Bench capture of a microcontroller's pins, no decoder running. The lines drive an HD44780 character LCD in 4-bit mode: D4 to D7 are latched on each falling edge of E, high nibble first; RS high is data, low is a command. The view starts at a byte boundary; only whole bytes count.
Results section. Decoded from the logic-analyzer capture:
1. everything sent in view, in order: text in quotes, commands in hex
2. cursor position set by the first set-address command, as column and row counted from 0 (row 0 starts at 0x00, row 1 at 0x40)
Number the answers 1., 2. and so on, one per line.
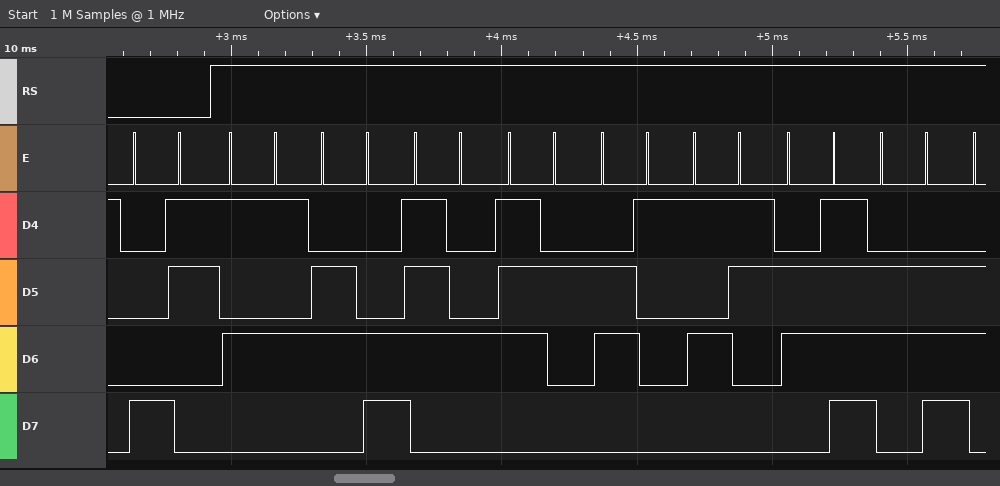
1. 0x83 "UltraSon"
2. column 3, row 0
